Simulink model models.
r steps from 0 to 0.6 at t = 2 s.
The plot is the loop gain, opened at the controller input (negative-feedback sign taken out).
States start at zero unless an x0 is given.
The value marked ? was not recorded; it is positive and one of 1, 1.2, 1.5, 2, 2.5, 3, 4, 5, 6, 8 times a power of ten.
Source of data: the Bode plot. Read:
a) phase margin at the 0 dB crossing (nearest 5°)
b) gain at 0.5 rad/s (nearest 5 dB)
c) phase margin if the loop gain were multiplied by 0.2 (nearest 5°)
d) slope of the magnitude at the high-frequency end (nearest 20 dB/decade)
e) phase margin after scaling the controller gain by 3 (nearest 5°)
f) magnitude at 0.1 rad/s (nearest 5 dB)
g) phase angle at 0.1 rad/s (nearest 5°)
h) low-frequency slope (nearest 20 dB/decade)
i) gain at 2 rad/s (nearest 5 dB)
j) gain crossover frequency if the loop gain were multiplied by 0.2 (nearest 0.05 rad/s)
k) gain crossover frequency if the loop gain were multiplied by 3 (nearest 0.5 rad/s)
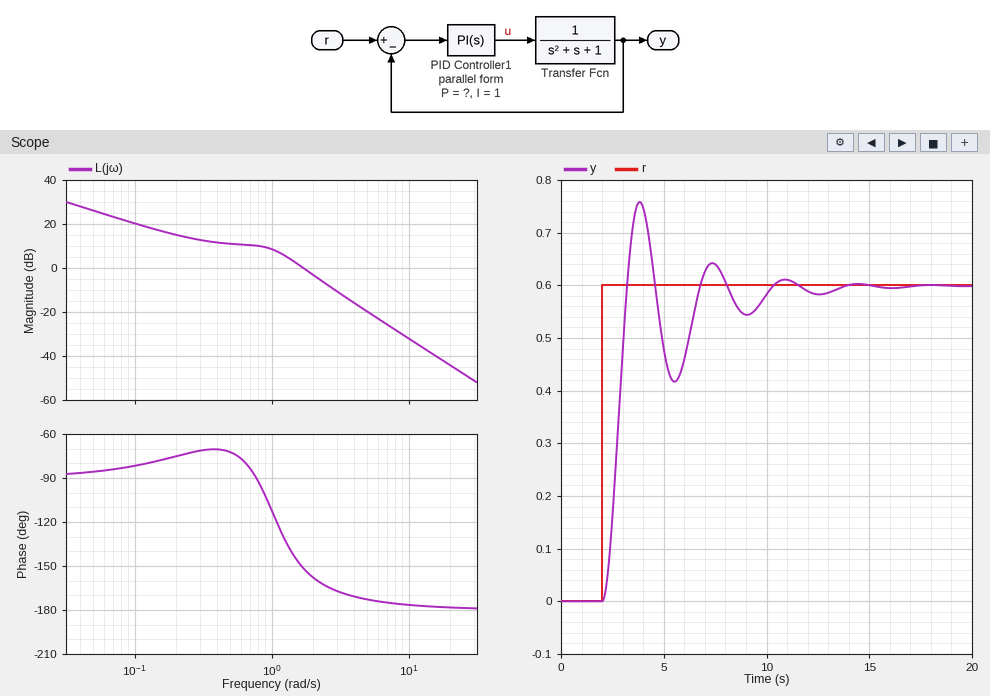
30°
10 dB
105°
-40 dB/decade
15°
20 dB
-80°
-20 dB/decade
-5 dB
0.25 rad/s
3.0 rad/s
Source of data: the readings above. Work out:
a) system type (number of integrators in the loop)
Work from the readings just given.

1
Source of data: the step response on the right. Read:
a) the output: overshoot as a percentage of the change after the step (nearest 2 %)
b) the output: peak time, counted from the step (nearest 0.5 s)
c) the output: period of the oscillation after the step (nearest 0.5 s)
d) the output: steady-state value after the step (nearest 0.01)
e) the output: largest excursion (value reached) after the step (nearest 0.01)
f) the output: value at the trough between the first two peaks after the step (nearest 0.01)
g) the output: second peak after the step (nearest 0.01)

26 %
2.0 s
3.5 s
0.60
0.76
0.42
0.64
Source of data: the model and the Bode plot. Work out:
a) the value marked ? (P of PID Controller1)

2.5
